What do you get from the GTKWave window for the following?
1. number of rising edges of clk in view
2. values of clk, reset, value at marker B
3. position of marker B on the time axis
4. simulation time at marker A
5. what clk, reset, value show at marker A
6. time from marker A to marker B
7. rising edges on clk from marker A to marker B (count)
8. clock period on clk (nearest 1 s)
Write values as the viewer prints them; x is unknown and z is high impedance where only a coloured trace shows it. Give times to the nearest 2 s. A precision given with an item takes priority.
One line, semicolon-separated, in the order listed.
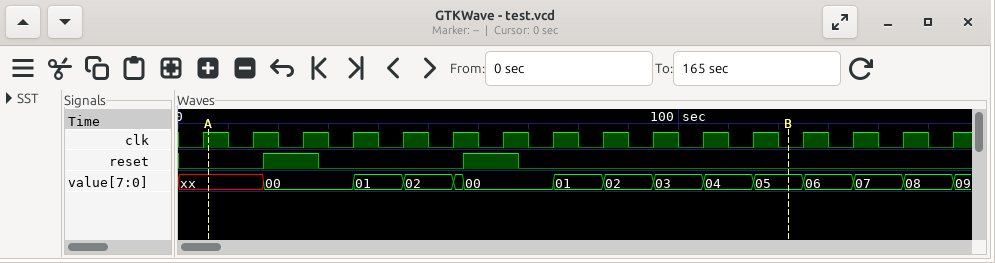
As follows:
16; clk=0, reset=0, value=05; 122 s; 6 s; clk=1, reset=0, value=xx; 116 s; 11; 10 s
